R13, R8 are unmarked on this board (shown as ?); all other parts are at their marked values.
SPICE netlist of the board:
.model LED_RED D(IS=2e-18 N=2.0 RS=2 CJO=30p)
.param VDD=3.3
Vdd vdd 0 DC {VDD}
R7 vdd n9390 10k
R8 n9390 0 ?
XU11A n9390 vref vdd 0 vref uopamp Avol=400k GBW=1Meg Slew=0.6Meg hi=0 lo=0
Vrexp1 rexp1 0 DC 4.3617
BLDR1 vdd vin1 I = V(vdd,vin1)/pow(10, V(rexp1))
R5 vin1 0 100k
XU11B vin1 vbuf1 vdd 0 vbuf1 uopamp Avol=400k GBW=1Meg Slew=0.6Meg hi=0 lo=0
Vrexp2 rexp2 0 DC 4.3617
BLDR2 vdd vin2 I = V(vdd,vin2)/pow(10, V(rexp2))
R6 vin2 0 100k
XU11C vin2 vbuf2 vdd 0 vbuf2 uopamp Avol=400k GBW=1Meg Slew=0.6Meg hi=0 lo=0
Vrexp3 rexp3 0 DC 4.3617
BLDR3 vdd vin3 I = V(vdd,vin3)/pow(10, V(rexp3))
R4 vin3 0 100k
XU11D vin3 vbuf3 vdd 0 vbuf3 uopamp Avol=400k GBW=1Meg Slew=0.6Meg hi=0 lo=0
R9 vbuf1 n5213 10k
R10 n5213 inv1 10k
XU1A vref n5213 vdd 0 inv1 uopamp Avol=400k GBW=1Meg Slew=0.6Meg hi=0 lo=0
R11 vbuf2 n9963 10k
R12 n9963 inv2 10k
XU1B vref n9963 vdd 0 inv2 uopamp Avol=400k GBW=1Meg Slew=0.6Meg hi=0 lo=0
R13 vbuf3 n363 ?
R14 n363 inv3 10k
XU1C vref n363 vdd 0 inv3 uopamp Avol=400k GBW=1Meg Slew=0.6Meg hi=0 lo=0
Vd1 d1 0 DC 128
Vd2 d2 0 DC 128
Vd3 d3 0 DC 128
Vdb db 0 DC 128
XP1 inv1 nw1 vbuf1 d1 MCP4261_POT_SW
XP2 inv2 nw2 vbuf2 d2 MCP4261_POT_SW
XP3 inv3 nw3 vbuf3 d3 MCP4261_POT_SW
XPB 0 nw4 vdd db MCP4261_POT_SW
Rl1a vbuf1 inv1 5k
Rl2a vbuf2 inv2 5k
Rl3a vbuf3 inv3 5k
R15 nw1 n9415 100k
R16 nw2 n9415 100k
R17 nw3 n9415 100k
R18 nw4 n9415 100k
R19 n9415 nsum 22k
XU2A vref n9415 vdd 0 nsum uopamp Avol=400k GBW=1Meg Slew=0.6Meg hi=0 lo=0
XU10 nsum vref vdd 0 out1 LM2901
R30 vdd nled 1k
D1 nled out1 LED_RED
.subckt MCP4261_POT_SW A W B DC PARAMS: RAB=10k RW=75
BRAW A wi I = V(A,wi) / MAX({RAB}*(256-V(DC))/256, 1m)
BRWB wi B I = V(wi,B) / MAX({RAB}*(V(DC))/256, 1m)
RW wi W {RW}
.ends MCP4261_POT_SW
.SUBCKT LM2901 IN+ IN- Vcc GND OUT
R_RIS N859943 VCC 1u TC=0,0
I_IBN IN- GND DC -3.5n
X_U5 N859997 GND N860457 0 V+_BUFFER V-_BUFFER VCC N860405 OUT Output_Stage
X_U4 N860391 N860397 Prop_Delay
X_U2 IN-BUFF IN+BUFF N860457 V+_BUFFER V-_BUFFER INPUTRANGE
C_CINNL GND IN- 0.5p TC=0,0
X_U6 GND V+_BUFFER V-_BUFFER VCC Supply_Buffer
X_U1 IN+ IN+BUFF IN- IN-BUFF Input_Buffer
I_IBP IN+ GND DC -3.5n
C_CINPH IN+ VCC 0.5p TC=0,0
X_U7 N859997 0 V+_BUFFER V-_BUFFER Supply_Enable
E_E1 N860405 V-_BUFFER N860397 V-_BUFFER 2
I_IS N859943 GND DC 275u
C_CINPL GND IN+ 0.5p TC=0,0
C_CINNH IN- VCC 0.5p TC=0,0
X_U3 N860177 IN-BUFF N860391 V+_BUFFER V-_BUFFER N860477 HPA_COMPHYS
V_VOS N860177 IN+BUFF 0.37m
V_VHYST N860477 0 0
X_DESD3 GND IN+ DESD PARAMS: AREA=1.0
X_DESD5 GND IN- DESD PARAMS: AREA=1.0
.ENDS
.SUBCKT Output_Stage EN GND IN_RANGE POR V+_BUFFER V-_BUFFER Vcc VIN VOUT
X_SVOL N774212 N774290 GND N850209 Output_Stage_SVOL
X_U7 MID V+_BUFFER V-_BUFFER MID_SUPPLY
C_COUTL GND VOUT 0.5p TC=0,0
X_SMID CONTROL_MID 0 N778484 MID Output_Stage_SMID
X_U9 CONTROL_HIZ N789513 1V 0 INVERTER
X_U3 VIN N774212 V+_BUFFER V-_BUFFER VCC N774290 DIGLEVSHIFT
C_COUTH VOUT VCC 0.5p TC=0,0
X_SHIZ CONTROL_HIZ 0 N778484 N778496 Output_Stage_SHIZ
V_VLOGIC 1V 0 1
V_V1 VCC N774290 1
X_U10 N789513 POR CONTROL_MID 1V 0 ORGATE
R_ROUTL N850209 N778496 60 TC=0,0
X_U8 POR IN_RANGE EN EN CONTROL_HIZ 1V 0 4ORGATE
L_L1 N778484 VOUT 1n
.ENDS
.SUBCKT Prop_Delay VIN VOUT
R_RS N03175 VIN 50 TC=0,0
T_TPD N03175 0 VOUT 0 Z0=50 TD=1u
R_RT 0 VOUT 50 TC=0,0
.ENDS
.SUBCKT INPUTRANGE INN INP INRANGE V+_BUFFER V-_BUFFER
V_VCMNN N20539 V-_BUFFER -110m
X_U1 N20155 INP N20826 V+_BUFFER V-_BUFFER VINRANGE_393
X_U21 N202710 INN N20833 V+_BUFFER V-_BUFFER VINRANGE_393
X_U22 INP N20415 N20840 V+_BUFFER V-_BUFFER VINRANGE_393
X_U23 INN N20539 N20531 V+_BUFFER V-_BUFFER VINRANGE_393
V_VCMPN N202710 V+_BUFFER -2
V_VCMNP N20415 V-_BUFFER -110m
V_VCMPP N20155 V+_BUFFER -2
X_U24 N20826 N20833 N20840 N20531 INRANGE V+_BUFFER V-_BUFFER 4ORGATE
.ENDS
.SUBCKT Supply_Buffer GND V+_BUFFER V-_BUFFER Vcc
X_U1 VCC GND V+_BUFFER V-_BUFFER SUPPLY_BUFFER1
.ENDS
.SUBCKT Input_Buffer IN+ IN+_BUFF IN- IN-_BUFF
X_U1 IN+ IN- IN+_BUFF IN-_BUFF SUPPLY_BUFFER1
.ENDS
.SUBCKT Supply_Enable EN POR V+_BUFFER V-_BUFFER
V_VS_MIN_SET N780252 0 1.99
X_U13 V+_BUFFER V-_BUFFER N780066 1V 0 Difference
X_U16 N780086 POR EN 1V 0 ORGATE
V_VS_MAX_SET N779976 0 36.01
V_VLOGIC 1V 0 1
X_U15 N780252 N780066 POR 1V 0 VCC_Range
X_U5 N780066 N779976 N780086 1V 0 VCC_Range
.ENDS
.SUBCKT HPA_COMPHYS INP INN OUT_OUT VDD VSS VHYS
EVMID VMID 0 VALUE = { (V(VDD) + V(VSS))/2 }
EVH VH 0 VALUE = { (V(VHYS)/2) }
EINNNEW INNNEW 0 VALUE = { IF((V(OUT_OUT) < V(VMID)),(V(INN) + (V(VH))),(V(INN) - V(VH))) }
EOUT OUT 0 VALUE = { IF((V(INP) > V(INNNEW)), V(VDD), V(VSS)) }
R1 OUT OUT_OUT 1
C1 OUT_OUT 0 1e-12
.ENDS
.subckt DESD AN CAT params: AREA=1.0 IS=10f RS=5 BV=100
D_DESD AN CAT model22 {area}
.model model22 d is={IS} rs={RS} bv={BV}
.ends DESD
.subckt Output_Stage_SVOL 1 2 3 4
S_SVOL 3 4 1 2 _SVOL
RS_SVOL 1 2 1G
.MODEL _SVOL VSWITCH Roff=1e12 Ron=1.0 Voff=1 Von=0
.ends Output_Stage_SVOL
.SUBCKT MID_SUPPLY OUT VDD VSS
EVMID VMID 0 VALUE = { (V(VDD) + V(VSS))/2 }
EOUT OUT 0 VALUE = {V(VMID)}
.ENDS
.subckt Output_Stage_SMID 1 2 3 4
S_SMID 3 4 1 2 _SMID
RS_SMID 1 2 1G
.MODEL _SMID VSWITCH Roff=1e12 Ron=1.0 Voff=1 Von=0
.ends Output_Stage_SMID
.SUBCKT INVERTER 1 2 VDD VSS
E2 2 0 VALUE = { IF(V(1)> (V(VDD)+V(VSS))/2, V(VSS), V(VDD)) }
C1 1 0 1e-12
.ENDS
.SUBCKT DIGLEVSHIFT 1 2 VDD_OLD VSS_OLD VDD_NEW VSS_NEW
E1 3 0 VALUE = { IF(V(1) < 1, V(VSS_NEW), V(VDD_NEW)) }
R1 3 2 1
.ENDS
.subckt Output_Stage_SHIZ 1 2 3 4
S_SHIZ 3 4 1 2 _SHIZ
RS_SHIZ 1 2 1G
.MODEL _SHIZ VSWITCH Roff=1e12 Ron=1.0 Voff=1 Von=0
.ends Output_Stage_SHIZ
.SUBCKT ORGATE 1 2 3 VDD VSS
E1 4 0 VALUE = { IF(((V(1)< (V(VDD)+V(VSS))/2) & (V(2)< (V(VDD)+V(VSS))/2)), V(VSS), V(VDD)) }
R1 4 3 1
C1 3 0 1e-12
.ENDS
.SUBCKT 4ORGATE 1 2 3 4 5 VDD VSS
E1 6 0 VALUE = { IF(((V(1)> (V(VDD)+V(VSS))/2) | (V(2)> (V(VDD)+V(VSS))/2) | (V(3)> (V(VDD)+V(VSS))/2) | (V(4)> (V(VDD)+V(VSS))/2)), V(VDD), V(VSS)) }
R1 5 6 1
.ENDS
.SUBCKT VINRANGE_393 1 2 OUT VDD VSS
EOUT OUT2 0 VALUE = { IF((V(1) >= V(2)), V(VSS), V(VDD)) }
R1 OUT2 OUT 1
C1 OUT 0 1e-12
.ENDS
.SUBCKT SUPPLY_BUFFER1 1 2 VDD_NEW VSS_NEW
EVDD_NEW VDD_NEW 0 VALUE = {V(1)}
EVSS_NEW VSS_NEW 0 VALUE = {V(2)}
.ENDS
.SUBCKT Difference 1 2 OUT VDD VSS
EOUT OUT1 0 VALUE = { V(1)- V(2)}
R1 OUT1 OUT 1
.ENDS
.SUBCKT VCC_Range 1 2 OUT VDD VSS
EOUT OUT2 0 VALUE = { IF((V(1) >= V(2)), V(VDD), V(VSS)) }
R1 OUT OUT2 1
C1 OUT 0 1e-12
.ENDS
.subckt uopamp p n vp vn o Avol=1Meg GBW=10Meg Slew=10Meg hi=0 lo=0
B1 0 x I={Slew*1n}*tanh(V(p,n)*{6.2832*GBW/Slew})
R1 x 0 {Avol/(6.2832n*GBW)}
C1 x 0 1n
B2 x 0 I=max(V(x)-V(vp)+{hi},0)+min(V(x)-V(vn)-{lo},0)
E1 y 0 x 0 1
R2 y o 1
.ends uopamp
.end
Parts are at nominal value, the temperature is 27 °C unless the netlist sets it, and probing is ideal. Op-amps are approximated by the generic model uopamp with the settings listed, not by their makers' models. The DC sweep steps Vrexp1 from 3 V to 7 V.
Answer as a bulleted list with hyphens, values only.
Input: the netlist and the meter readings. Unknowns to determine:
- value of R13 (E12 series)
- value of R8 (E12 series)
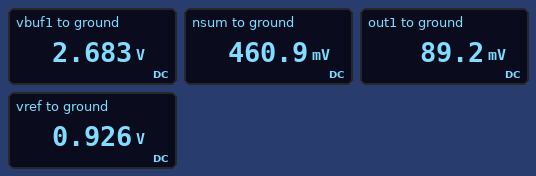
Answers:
- 33 kΩ
- 3.9 kΩ
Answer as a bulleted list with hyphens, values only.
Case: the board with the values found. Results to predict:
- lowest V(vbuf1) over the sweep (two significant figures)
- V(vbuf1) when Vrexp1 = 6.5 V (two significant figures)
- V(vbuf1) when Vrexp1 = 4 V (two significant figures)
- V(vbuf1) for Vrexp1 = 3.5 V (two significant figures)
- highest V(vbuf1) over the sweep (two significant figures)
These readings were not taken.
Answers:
- 33 mV
- 100 mV
- 3.0 V
- 3.2 V
- 3.3 V
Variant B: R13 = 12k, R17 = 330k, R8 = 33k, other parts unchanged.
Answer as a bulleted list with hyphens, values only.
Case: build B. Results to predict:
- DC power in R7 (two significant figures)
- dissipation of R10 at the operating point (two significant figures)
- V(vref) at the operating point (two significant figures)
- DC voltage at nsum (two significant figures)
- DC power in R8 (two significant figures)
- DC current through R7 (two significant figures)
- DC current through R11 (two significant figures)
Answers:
- 59 µW
- 2.3 µW
- 2.5 V
- 2.7 V
- 190 µW
- 77 µA
- 15 µA
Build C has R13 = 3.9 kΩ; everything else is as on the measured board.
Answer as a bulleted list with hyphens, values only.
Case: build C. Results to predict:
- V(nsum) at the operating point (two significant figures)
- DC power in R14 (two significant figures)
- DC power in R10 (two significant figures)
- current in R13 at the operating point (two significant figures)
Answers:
- 500 mV
- 370 µW
- 180 µW
- 190 µA
